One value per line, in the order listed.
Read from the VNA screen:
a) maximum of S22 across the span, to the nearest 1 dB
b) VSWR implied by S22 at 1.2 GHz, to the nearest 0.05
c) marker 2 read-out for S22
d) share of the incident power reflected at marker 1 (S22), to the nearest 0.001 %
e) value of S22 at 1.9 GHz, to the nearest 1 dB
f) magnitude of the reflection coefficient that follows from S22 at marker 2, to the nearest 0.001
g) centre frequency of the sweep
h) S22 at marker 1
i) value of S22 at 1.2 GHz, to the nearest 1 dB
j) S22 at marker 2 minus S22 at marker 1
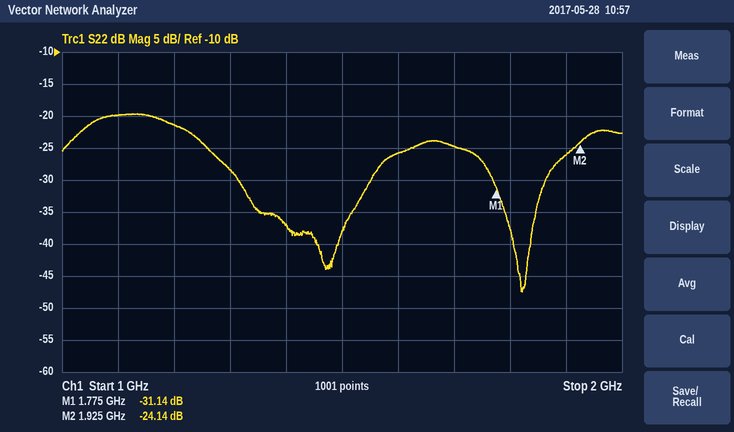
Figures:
-20 dB
1.20
-24.14 dB
0.077 %
-26 dB
0.062
1.5 GHz
-31.14 dB
-21 dB
7.00 dB
